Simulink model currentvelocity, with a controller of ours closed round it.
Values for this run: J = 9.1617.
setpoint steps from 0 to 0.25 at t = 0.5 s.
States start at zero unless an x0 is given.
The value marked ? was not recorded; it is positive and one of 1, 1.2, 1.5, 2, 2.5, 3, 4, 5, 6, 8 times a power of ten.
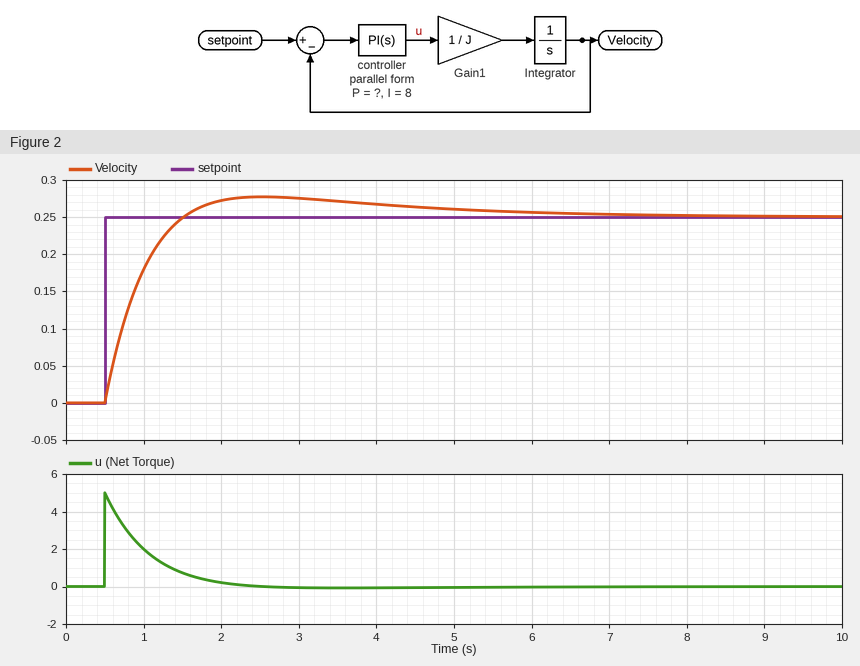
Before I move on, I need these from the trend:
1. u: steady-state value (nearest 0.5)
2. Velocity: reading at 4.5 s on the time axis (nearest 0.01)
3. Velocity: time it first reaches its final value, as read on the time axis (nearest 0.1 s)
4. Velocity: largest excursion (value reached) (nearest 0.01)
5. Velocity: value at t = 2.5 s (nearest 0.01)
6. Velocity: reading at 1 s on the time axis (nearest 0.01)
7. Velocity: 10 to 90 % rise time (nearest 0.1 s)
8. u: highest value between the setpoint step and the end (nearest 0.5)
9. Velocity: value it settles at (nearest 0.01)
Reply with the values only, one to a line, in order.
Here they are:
0.0
0.26
1.5 s
0.28
0.28
0.18
0.7 s
5.0
0.25
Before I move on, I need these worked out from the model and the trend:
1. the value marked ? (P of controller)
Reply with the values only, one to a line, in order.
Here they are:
20
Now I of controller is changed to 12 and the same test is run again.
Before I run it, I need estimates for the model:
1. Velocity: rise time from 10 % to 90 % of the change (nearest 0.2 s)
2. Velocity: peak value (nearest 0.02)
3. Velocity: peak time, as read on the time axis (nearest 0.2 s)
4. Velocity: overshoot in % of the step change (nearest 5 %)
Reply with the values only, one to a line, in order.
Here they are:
0.6 s
0.28
2.2 s
15 %
